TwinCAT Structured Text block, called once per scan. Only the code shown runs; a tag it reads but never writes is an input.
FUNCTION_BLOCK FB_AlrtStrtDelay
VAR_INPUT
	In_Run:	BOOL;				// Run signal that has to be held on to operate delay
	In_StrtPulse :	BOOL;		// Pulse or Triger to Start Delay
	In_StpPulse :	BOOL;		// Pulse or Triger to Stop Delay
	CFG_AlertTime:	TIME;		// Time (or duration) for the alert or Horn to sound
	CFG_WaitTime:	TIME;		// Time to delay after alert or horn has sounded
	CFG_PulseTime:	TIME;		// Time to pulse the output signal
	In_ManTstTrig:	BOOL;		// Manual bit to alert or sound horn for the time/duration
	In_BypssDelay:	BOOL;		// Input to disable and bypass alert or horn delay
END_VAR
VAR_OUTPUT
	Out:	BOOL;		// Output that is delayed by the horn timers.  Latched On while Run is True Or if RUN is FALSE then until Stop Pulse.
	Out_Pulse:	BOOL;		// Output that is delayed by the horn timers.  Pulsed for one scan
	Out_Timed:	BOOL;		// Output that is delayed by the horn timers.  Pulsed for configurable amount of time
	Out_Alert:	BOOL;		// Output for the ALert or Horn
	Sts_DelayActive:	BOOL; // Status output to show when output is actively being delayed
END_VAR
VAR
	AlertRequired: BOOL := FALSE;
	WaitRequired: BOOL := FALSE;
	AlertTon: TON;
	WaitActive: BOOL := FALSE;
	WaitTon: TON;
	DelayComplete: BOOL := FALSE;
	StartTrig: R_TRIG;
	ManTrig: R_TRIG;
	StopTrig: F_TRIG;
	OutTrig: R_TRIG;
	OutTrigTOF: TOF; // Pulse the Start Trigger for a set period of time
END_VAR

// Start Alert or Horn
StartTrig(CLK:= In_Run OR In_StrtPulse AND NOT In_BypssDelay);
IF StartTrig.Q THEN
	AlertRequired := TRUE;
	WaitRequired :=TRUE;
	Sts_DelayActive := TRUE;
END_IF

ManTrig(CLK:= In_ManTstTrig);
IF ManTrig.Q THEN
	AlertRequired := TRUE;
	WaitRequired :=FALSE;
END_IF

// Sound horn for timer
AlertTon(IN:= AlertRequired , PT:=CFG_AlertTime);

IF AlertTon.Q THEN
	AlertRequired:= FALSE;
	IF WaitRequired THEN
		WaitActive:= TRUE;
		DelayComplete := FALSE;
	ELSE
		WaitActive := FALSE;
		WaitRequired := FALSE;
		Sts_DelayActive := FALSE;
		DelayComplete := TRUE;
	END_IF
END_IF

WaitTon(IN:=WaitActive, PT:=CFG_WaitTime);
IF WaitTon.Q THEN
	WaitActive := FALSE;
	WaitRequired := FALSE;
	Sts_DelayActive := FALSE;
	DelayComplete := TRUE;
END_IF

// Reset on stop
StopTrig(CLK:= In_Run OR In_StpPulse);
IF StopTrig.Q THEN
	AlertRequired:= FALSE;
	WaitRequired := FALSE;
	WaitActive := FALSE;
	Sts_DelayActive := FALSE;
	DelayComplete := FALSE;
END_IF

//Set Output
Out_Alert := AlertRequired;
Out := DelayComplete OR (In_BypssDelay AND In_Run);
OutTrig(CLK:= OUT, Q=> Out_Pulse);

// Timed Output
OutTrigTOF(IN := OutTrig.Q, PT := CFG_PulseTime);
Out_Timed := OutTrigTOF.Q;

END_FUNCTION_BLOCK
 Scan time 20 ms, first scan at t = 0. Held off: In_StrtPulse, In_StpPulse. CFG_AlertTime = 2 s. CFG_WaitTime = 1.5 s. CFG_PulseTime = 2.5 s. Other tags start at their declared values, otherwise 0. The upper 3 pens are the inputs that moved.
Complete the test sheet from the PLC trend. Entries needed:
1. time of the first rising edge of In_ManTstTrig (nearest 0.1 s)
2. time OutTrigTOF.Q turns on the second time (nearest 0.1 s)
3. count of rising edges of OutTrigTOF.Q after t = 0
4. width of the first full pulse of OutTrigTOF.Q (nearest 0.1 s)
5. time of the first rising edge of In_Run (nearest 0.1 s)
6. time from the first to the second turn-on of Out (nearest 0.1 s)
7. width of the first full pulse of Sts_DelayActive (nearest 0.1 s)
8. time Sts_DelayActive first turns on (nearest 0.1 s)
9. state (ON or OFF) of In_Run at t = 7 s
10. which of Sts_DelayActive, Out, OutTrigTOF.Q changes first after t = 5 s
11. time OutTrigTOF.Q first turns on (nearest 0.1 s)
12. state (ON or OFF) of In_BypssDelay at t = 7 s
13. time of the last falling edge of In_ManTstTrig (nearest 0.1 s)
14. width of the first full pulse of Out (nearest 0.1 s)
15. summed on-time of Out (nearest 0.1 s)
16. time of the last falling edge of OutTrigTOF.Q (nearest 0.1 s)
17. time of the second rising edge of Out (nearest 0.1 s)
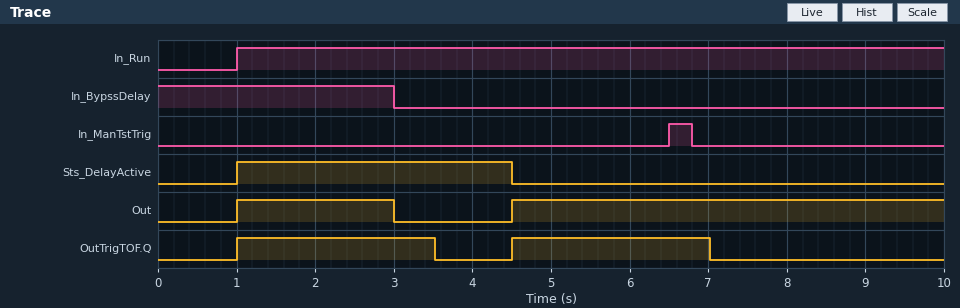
6.5 s
4.5 s
2
2.5 s
1.0 s
3.5 s
3.5 s
1.0 s
ON
OutTrigTOF.Q
1.0 s
OFF
6.8 s
2.0 s
7.5 s
7.0 s
4.5 s
